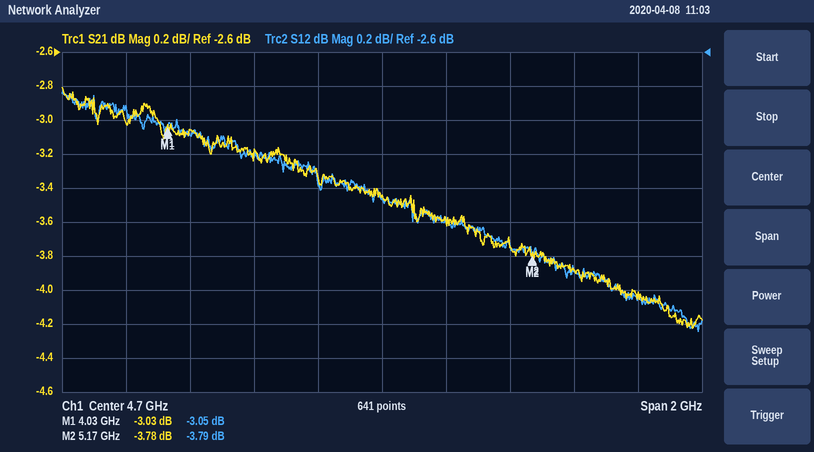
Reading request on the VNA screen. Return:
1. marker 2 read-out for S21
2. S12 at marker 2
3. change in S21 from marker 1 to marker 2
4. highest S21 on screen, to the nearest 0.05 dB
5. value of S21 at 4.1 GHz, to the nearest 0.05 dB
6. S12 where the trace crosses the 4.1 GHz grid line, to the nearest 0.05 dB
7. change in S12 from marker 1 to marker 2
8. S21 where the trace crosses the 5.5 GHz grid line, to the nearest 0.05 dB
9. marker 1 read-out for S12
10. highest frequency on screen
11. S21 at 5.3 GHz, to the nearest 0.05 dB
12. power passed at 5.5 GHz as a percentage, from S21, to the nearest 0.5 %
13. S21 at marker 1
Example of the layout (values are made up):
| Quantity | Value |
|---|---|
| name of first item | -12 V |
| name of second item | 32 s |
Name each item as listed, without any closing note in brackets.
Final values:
| Quantity | Value |
|---|---|
| marker 2 read-out for S21 | -3.78 dB |
| S12 at marker 2 | -3.79 dB |
| change in S21 from marker 1 to marker 2 | -0.75 dB |
| highest S21 on screen, to the nearest 0.05 dB | -2.80 dB |
| value of S21 at 4.1 GHz, to the nearest 0.05 dB | -3.05 dB |
| S12 where the trace crosses the 4.1 GHz grid line, to the nearest 0.05 dB | -3.10 dB |
| change in S12 from marker 1 to marker 2 | -0.74 dB |
| S21 where the trace crosses the 5.5 GHz grid line, to the nearest 0.05 dB | -4.05 dB |
| marker 1 read-out for S12 | -3.05 dB |
| highest frequency on screen | 5.7 GHz |
| S21 at 5.3 GHz, to the nearest 0.05 dB | -3.90 dB |
| power passed at 5.5 GHz as a percentage, from S21, to the nearest 0.5 % | 39.5 % |
| S21 at marker 1 | -3.03 dB |
